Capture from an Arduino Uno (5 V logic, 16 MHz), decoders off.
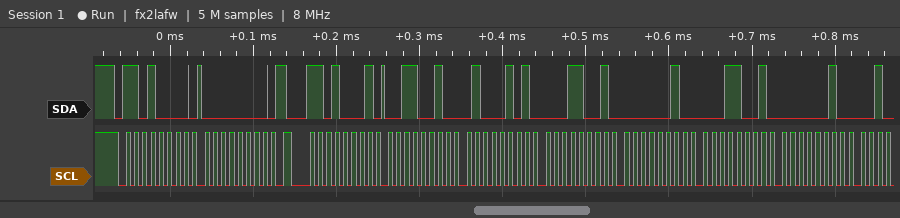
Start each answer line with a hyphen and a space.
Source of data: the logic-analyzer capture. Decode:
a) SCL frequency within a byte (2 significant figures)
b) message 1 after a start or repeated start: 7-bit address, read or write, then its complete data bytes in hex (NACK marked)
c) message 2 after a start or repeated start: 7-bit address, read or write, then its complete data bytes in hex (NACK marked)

- 100 kHz
- 0x68 write: 00
- 0x68 read: 32 45 19 02 19 02
